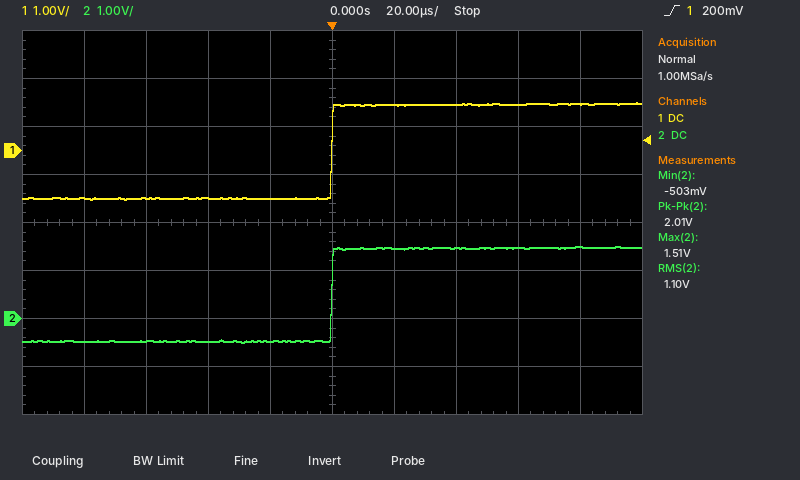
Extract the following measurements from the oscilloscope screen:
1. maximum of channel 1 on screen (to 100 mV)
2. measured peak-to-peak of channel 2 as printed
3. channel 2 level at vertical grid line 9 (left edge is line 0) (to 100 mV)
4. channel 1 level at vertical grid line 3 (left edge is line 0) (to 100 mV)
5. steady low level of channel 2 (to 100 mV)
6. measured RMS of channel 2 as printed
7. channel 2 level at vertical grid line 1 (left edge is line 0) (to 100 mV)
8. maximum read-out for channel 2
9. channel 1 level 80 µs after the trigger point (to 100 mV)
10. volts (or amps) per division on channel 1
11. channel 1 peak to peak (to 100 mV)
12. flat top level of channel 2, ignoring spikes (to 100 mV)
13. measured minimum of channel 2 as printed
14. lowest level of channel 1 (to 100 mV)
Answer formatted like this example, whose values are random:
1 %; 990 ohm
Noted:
1.0 V; 2.01 V; 1.5 V; -1.0 V; -500 mV; 1.10 V; -500 mV; 1.51 V; 1.0 V; 1 V; 2.0 V; 1.5 V; -503 mV; -1.0 V
